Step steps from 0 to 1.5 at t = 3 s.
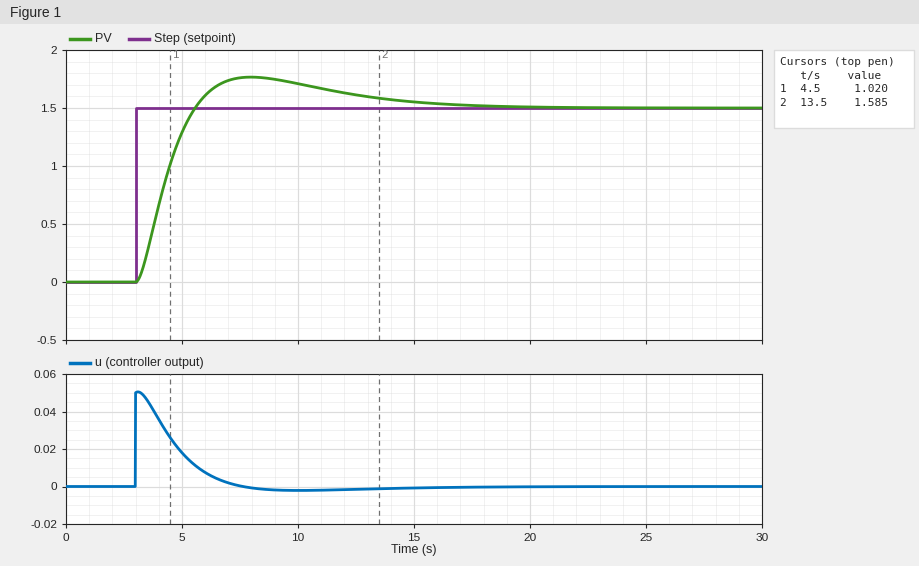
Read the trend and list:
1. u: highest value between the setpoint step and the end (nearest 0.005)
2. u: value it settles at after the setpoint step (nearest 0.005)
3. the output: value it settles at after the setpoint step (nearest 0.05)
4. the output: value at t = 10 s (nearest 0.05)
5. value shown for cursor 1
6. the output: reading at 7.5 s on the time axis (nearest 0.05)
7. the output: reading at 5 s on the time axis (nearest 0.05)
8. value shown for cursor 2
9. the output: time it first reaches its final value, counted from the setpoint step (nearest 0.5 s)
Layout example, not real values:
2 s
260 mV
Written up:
0.050
0.000
1.50
1.70
1.020
1.75
1.30
1.585
2.5 s
